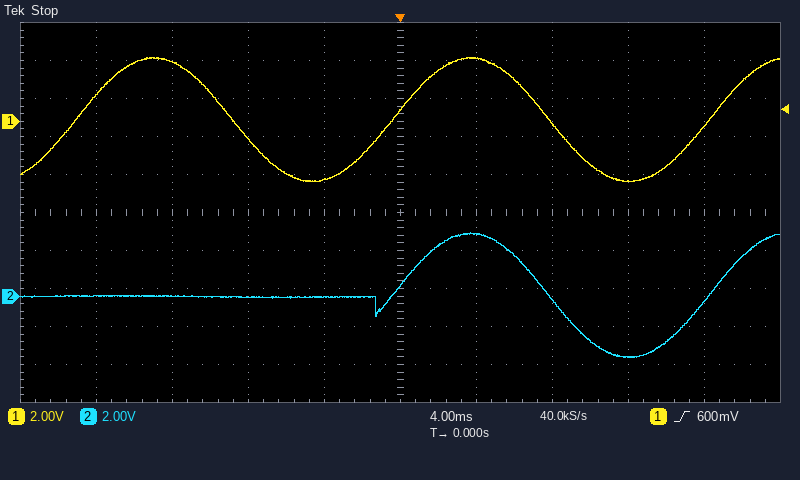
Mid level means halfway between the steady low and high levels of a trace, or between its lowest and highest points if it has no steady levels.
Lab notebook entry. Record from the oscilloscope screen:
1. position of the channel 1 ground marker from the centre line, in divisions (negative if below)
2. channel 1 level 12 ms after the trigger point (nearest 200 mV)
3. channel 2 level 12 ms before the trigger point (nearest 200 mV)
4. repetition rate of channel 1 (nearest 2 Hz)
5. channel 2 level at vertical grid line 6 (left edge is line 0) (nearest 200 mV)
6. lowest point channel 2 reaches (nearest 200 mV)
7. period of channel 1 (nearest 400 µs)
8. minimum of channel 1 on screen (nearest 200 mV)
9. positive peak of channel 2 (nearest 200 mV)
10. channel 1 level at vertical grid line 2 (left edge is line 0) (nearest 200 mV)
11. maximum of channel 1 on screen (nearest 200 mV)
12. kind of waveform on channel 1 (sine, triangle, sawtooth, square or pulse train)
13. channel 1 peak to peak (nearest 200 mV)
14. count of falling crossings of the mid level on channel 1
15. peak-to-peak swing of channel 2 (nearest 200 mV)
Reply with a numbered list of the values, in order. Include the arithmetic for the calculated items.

1. +2.4 div
2. -3.2 V
3. 0.0 V
4. 1 / 16.8 ms ≈ 60 Hz
5. 3.2 V
6. -3.2 V
7. 16.8 ms
8. -3.2 V
9. 3.4 V
10. 3.2 V
11. 3.4 V
12. sine
13. 3.4 V − (-3.2 V) = 6.6 V
14. 2
15. 3.4 V − (-3.2 V) = 6.6 V
